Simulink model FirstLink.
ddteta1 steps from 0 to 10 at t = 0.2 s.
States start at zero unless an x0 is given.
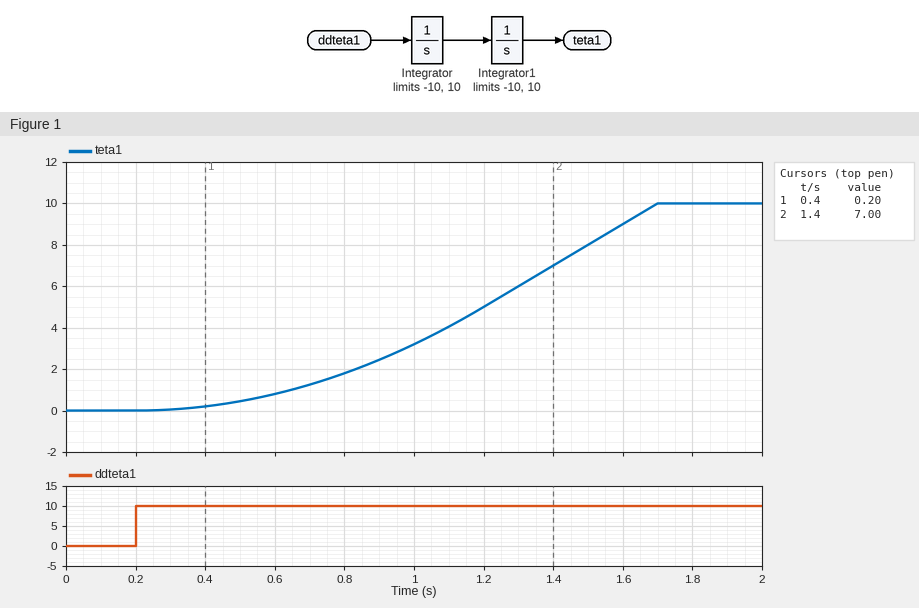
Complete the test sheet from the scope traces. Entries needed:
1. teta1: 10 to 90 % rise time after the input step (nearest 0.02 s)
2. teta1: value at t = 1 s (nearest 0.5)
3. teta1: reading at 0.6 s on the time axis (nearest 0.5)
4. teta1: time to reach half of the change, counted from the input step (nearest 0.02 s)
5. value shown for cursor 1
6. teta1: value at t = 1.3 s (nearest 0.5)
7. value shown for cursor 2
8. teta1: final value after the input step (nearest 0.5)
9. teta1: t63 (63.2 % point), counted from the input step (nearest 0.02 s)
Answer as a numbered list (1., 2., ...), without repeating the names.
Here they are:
1. 0.96 s
2. 3.0
3. 1.0
4. 1.00 s
5. 0.20
6. 6.0
7. 7.00
8. 10.0
9. 1.14 s
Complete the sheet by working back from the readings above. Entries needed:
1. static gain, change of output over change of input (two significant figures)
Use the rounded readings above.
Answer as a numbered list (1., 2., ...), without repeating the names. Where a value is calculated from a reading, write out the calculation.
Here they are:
1. (10 - 0) / (10 - 0) = 1.0
